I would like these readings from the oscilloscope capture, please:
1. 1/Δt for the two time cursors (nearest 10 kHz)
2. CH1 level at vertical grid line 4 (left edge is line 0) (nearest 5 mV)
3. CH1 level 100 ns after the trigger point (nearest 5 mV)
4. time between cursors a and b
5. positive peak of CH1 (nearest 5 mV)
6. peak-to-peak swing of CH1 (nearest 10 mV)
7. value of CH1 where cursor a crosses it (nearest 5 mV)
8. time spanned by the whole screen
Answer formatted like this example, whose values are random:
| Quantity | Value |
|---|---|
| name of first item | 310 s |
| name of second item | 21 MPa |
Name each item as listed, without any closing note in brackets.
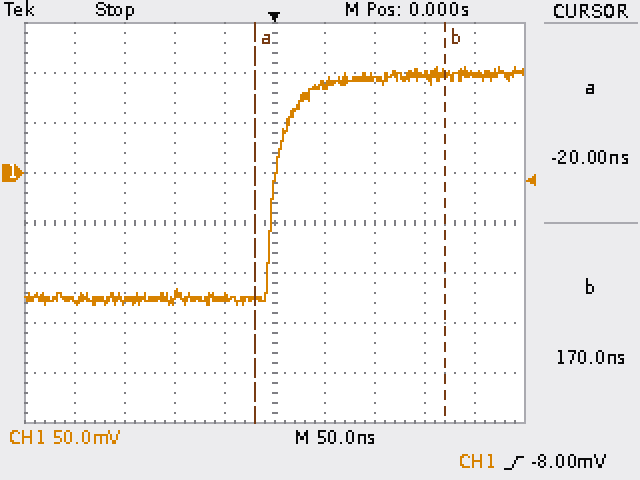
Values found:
| Quantity | Value |
|---|---|
| 1/Δt for the two time cursors | 5.26 MHz |
| CH1 level at vertical grid line 4 (left edge is line 0) | -125 mV |
| CH1 level 100 ns after the trigger point | 95 mV |
| time between cursors a and b | 190 ns |
| positive peak of CH1 | 105 mV |
| peak-to-peak swing of CH1 | 240 mV |
| value of CH1 where cursor a crosses it | -125 mV |
| time spanned by the whole screen | 500 ns |
